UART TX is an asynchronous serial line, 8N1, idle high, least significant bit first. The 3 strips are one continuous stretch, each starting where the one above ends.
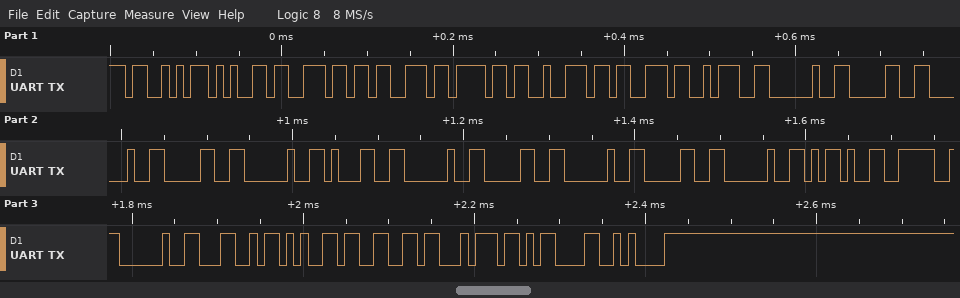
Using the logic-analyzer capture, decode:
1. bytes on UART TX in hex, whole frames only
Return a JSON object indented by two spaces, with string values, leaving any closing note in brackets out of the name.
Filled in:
{
  "bytes on UART TX in hex, whole frames only": "53 65 6E 73 6F 72 73 3A 20 30 20 30 20 31 20 30 20 30 20 2D 3E 20 4C 65 66 74 0D 0A"
}
